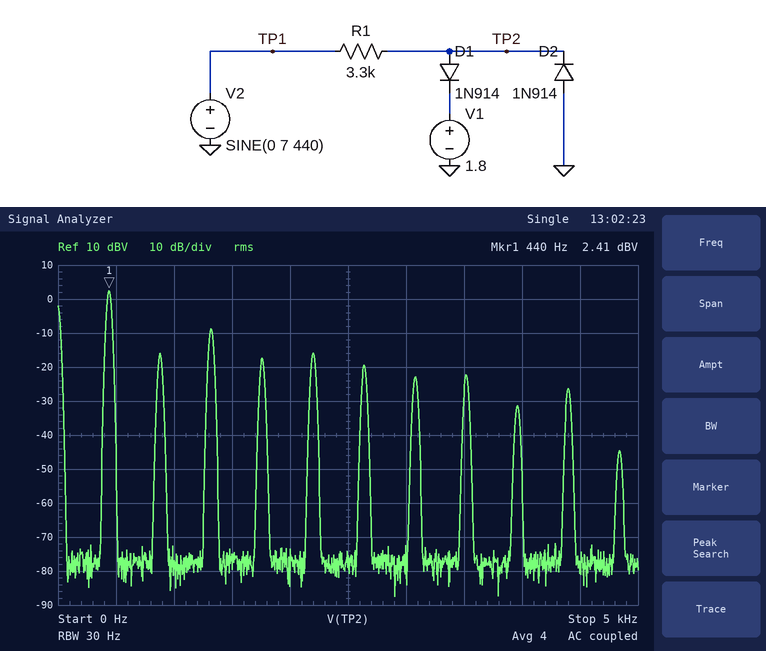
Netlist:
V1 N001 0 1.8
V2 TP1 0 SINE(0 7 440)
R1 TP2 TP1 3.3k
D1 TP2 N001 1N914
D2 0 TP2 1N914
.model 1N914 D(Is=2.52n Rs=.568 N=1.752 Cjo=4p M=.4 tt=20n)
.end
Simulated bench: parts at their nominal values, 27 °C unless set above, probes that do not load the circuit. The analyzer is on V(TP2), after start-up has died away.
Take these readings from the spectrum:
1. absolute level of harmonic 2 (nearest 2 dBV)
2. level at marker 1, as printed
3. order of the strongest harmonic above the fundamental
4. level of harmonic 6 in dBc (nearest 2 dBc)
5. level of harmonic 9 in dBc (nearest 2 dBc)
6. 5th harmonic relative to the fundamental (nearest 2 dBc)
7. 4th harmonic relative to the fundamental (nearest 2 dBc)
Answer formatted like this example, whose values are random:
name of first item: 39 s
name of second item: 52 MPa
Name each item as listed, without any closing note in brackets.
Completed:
absolute level of harmonic 2: -16 dBV
level at marker 1, as printed: 2.41 dBV
order of the strongest harmonic above the fundamental: 3
level of harmonic 6 in dBc: -22 dBc
level of harmonic 9 in dBc: -34 dBc
5th harmonic relative to the fundamental: -18 dBc
4th harmonic relative to the fundamental: -20 dBc
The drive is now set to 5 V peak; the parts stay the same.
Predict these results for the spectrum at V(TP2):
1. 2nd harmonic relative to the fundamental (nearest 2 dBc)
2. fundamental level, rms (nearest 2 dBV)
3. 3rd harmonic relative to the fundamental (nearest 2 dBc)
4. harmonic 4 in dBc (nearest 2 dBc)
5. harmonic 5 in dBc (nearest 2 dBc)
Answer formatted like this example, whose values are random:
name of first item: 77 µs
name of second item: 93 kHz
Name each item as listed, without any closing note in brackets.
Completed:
2nd harmonic relative to the fundamental: -16 dBc
fundamental level, rms: 2 dBV
3rd harmonic relative to the fundamental: -12 dBc
harmonic 4 in dBc: -18 dBc
harmonic 5 in dBc: -22 dBc
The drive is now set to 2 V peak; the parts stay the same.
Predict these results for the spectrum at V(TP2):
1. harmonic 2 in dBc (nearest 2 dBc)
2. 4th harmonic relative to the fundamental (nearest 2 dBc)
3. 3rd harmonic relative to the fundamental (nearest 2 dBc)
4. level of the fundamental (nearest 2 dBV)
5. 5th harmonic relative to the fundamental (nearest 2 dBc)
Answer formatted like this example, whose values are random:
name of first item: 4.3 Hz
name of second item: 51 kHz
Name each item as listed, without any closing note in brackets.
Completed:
harmonic 2 in dBc: -12 dBc
4th harmonic relative to the fundamental: -30 dBc
3rd harmonic relative to the fundamental: -24 dBc
level of the fundamental: 0 dBV
5th harmonic relative to the fundamental: -30 dBc
